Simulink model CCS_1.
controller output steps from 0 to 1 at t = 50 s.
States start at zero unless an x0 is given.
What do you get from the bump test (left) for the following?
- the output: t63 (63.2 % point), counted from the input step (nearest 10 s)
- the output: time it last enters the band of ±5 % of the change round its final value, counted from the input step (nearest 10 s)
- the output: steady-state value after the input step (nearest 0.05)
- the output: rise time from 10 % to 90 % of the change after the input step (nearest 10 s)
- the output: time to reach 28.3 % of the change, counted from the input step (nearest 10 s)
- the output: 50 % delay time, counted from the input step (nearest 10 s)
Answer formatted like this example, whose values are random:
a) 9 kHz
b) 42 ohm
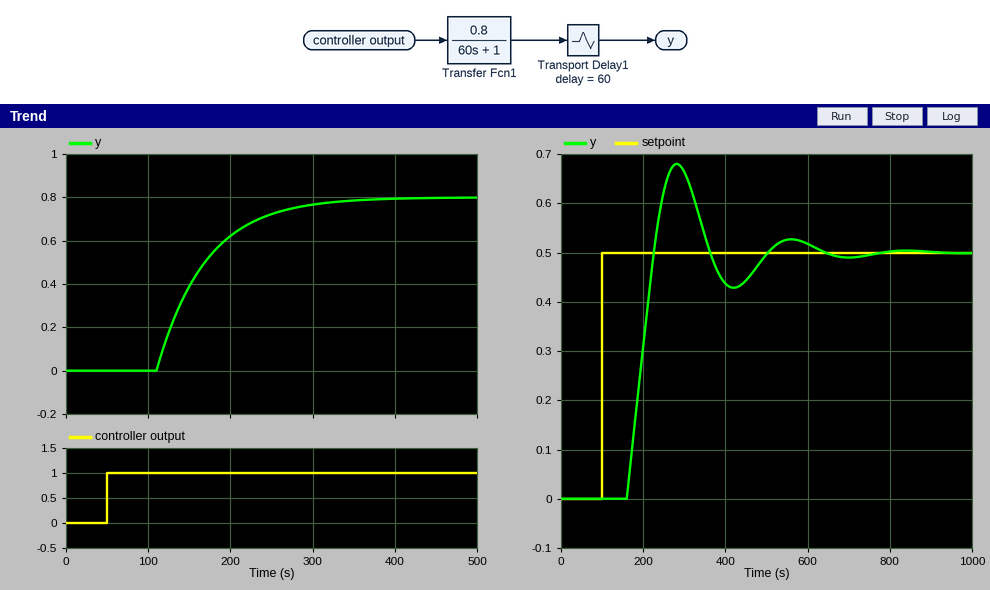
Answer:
a) 120 s
b) 240 s
c) 0.80
d) 130 s
e) 80 s
f) 100 s
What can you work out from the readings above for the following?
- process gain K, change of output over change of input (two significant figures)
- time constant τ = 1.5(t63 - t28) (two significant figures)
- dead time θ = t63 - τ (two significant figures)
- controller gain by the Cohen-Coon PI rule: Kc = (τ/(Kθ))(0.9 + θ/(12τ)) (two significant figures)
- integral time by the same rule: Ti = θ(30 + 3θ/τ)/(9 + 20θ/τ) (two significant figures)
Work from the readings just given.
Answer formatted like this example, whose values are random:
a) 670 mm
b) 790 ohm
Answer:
a) 0.80
b) 60 s
c) 60 s
d) 1.2
e) 68 s
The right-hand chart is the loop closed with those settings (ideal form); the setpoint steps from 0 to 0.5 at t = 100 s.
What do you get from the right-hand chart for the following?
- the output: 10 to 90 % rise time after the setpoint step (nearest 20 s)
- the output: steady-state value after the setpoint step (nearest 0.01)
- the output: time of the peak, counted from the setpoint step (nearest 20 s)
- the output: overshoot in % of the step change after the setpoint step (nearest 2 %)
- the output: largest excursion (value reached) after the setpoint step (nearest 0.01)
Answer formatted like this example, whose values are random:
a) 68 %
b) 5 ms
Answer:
a) 60 s
b) 0.50
c) 180 s
d) 36 %
e) 0.68
